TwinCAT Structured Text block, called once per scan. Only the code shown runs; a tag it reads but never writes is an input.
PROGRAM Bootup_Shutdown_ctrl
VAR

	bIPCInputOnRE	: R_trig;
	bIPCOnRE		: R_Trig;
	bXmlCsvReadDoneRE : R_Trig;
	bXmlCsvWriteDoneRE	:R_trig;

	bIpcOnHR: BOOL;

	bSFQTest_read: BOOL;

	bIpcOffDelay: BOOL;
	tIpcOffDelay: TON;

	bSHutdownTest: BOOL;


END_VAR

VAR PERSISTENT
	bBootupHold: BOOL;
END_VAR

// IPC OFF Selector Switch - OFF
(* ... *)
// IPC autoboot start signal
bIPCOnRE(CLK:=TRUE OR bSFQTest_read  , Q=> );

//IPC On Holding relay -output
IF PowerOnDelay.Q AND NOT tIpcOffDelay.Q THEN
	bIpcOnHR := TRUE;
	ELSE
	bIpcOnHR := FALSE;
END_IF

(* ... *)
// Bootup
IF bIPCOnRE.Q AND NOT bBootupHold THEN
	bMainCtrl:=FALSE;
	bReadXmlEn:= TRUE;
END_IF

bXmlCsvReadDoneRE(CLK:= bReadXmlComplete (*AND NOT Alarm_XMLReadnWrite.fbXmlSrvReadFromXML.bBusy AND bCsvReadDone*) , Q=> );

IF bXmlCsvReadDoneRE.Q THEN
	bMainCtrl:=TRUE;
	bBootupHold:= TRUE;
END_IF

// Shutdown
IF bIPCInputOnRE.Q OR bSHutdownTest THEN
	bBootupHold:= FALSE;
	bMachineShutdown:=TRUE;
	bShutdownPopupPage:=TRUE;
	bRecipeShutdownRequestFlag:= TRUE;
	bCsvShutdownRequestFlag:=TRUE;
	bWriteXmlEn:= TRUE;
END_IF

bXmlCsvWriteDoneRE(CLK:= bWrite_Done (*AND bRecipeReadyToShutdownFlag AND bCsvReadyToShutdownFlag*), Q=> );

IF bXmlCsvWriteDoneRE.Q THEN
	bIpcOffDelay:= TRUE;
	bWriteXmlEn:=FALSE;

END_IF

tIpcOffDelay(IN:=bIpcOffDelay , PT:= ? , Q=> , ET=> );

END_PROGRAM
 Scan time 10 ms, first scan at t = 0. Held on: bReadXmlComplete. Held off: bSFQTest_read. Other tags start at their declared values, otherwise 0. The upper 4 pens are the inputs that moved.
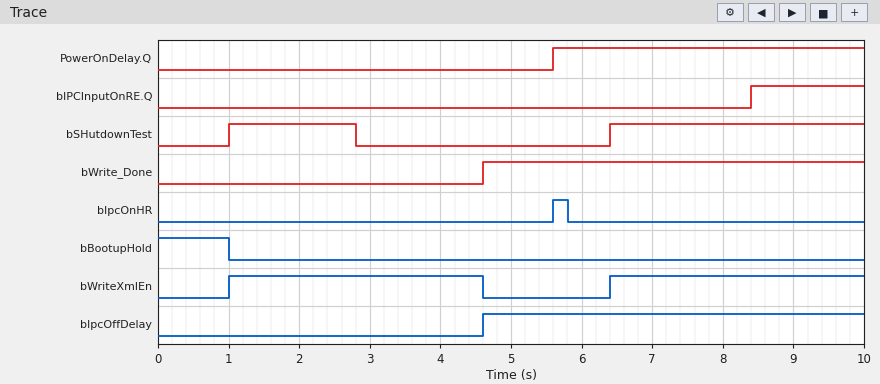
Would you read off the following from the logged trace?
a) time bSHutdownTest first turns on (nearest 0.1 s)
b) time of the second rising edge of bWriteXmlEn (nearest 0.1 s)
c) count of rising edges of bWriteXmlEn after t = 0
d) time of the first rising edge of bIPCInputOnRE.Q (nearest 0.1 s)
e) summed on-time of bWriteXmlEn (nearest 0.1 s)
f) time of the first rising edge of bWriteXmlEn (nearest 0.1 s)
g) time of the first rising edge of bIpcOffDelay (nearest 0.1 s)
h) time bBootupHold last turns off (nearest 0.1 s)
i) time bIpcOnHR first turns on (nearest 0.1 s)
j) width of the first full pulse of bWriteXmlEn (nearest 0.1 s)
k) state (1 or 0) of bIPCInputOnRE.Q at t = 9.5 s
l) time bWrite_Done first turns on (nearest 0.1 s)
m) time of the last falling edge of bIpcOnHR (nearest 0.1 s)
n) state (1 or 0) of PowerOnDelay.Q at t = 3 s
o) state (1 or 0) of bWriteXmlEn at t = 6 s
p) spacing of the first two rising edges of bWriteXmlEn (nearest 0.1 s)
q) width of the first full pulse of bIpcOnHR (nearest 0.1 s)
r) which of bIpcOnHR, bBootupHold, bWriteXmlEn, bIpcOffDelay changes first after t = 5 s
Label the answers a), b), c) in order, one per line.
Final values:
a) 1.0 s
b) 6.4 s
c) 2
d) 8.4 s
e) 7.2 s
f) 1.0 s
g) 4.6 s
h) 1.0 s
i) 5.6 s
j) 3.6 s
k) 1
l) 4.6 s
m) 5.8 s
n) 0
o) 0
p) 5.4 s
q) 0.2 s
r) bIpcOnHR
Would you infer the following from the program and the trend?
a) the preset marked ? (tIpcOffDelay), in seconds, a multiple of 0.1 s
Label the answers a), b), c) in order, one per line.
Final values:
a) 1.2 s
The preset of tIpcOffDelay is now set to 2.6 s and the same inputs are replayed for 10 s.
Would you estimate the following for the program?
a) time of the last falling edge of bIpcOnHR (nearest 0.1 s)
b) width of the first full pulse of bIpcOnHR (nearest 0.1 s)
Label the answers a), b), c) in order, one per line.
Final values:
a) 7.2 s
b) 1.6 s
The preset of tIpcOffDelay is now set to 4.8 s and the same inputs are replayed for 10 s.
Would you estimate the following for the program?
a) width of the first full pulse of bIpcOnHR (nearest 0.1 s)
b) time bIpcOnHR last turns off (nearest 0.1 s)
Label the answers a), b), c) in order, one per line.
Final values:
a) 3.8 s
b) 9.4 s
